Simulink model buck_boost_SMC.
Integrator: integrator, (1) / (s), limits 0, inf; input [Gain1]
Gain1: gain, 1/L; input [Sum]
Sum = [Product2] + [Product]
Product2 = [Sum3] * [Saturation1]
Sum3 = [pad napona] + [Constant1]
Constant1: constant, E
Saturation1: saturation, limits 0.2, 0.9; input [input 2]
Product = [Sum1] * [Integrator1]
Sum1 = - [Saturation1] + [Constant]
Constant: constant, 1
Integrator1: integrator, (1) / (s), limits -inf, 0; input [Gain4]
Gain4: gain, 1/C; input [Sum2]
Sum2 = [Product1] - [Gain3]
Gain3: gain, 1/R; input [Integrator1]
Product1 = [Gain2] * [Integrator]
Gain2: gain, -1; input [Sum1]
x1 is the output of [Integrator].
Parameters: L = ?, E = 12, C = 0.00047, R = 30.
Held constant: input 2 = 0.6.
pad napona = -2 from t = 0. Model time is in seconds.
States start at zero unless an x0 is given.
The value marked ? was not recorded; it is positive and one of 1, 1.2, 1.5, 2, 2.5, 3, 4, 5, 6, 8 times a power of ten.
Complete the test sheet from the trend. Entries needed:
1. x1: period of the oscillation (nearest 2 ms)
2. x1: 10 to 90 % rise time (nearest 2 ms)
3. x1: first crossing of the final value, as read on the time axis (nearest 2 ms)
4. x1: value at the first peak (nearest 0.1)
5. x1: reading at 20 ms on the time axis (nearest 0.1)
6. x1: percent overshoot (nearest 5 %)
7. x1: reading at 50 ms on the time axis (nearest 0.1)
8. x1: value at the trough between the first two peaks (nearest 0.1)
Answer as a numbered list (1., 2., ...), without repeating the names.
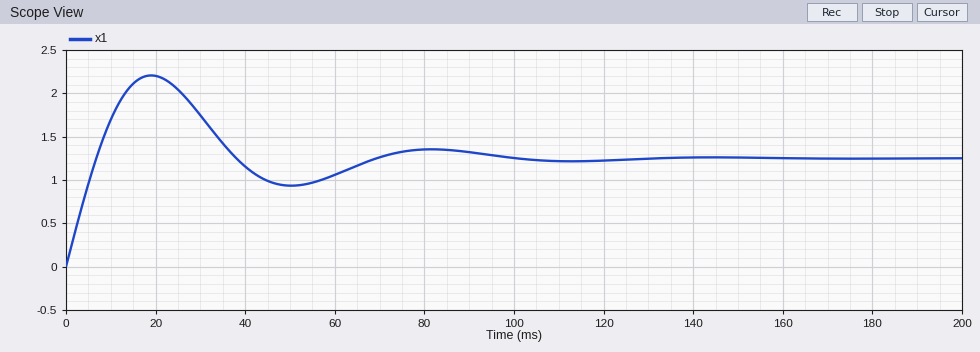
1. 62 ms
2. 6 ms
3. 6 ms
4. 2.2
5. 2.2
6. 75 %
7. 0.9
8. 0.9
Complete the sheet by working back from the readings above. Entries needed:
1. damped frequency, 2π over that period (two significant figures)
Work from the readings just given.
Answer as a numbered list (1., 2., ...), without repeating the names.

1. 0.10 rad/ms
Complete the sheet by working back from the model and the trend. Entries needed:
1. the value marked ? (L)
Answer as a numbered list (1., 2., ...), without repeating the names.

1. 0.03
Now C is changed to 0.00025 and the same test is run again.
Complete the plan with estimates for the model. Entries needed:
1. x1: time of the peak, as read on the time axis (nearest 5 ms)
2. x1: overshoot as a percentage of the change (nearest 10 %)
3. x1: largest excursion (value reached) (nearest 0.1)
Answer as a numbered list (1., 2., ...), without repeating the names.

1. 15 ms
2. 40 %
3. 1.7
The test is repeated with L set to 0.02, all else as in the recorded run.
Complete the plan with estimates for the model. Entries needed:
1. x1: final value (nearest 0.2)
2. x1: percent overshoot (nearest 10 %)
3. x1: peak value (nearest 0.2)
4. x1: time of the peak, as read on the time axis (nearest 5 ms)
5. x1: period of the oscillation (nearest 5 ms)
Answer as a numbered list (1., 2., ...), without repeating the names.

1. 1.2
2. 110 %
3. 2.6
4. 15 ms
5. 50 ms
